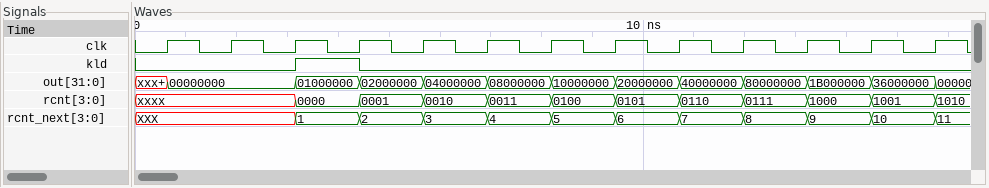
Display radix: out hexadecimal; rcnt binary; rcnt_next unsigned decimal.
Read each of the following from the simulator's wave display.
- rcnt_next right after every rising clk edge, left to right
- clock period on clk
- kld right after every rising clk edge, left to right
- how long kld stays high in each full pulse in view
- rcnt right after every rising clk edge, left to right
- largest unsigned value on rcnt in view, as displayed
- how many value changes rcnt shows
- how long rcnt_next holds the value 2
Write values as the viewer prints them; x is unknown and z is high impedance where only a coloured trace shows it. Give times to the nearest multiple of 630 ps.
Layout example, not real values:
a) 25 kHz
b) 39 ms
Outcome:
a) XXX, XXX, 1, 2, 3, 4, 5, 6, 7, 8, 9, 10, 11
b) 1260 ps
c) 0 0 1 0 0 0 0 0 0 0 0 0 0
d) 1260 ps
e) xxxx, xxxx, 0000, 0001, 0010, 0011, 0100, 0101, 0110, 0111, 1000, 1001, 1010
f) 1010
g) 11
h) 1260 ps
